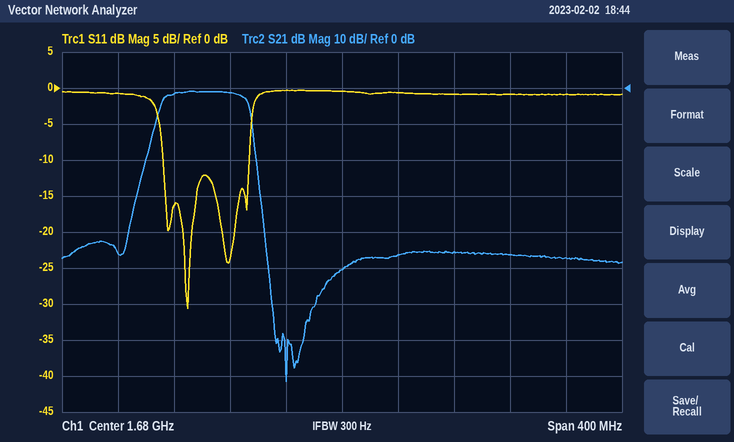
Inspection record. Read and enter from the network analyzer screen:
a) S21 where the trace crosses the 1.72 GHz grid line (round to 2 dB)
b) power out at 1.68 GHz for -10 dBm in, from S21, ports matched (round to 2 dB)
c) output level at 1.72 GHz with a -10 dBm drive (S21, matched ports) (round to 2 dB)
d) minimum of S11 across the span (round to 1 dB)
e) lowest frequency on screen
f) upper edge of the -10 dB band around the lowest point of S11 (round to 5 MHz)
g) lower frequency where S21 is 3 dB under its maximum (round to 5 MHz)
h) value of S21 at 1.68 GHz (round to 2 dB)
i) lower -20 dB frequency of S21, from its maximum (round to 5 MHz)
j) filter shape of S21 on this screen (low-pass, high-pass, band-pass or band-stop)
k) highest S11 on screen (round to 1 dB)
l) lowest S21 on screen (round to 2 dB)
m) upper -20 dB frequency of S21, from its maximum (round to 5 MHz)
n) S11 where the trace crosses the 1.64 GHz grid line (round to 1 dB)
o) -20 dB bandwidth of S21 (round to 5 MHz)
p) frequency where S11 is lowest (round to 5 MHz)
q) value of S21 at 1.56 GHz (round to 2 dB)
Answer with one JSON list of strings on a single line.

["-46 dB", "-60 dBm", "-56 dBm", "-31 dB", "1.48 GHz", "1.615 GHz", "1.550 GHz", "-50 dB", "1.540 GHz", "band-pass", "0 dB", "-82 dB", "1.620 GHz", "0 dB", "80 MHz", "1.570 GHz", "-2 dB"]
